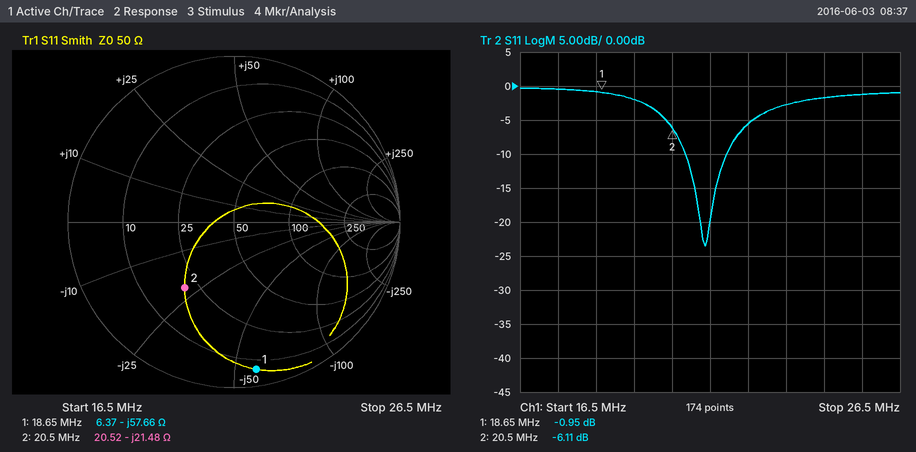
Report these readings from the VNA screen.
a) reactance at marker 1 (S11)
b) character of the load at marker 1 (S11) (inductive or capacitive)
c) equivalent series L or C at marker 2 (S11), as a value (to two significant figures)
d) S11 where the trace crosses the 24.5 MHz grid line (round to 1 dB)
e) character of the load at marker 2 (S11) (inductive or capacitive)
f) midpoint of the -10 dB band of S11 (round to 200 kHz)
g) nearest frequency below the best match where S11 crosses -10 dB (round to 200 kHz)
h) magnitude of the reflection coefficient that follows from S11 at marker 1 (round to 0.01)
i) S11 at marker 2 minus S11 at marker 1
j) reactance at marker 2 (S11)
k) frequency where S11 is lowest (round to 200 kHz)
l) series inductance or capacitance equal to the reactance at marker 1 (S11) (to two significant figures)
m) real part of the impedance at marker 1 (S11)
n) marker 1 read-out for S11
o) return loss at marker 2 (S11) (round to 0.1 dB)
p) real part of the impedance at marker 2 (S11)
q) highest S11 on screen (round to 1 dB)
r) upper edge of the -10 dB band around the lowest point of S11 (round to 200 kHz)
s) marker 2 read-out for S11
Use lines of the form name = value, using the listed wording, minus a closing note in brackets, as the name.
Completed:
reactance at marker 1 = -57.66 Ω
character of the load at marker 1 (S11) = capacitive
equivalent series L or C at marker 2 (S11), as a value = 360 pF
S11 where the trace crosses the 24.5 MHz grid line = -2 dB
character of the load at marker 2 (S11) = capacitive
midpoint of the -10 dB band of S11 = 21.4 MHz
nearest frequency below the best match where S11 crosses -10 dB = 20.8 MHz
magnitude of the reflection coefficient that follows from S11 at marker 1 = 0.90
S11 at marker 2 minus S11 at marker 1 = -5.16 dB
reactance at marker 2 = -21.48 Ω
frequency where S11 is lowest = 21.4 MHz
series inductance or capacitance equal to the reactance at marker 1 (S11) = 150 pF
real part of the impedance at marker 1 = 6.37 Ω
marker 1 read-out for S11 = -0.95 dB
return loss at marker 2 (S11) = 6.1 dB
real part of the impedance at marker 2 = 20.52 Ω
highest S11 on screen = 0 dB
upper edge of the -10 dB band around the lowest point of S11 = 22.0 MHz
marker 2 read-out for S11 = -6.11 dB
